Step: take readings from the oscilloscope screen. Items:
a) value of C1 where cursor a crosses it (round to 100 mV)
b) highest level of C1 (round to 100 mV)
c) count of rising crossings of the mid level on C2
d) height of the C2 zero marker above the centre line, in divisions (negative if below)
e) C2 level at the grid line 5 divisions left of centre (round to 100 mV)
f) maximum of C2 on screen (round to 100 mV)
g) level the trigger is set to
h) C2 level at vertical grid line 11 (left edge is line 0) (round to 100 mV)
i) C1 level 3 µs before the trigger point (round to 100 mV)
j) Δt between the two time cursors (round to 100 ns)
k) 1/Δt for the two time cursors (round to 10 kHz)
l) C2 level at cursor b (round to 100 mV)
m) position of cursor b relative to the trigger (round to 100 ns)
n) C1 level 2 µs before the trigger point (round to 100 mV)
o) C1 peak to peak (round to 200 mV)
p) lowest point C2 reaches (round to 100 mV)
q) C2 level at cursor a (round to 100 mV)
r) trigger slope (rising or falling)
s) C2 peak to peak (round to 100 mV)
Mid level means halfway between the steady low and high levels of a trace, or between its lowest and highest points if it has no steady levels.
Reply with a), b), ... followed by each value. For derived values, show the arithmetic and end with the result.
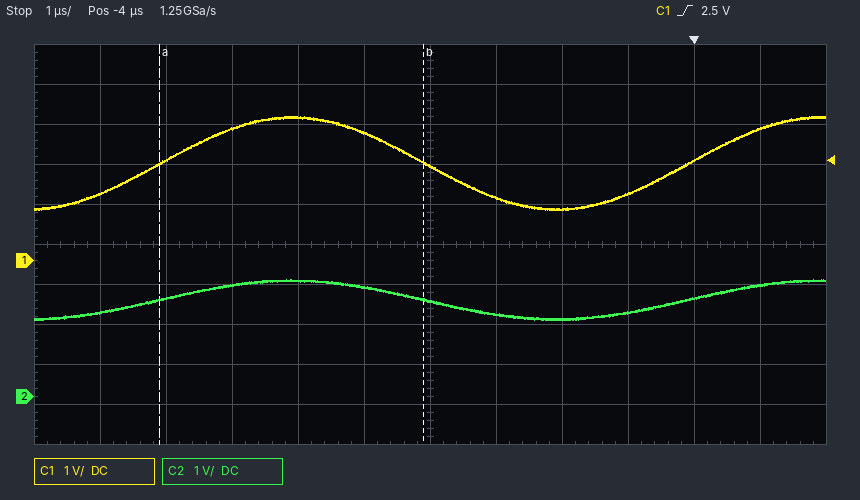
a) 2.4 V
b) 3.6 V
c) 2
d) -3.8 div
e) 2.1 V
f) 2.9 V
g) 2.5 V
h) 2.8 V
i) 1.6 V
j) 4.0 µs
k) 1 / 4.0 µs ≈ 250 kHz
l) 2.4 V
m) -4.1 µs
n) 1.3 V
o) 2.4 V
p) 1.9 V
q) 2.4 V
r) rising
s) 2.9 V − (1.9 V) = 1.0 V
